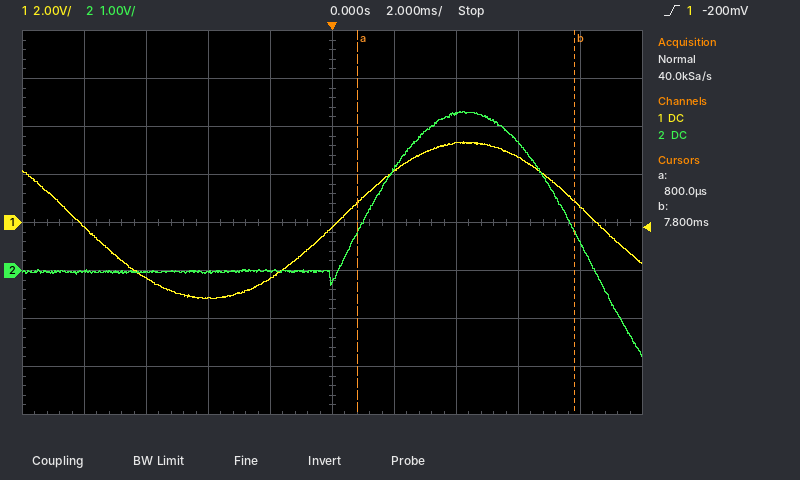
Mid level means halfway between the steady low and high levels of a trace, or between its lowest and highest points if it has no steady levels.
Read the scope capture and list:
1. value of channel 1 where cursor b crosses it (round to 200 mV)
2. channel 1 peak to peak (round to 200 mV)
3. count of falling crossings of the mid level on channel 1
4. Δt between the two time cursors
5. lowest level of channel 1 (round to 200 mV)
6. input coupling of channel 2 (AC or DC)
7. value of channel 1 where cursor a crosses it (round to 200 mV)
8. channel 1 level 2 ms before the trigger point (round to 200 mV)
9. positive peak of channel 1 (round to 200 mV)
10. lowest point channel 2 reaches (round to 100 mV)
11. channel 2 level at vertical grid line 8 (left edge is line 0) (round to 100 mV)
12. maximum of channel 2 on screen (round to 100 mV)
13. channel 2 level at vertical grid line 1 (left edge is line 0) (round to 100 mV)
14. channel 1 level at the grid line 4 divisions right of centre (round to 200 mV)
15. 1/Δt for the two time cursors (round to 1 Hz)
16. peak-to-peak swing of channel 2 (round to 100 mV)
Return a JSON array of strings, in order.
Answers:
["800 mV", "6.6 V", "2", "7.0 ms", "-3.2 V", "DC", "800 mV", "-2.4 V", "3.4 V", "-1.8 V", "2.7 V", "3.3 V", "0.0 V", "600 mV", "143 Hz", "5.1 V"]
